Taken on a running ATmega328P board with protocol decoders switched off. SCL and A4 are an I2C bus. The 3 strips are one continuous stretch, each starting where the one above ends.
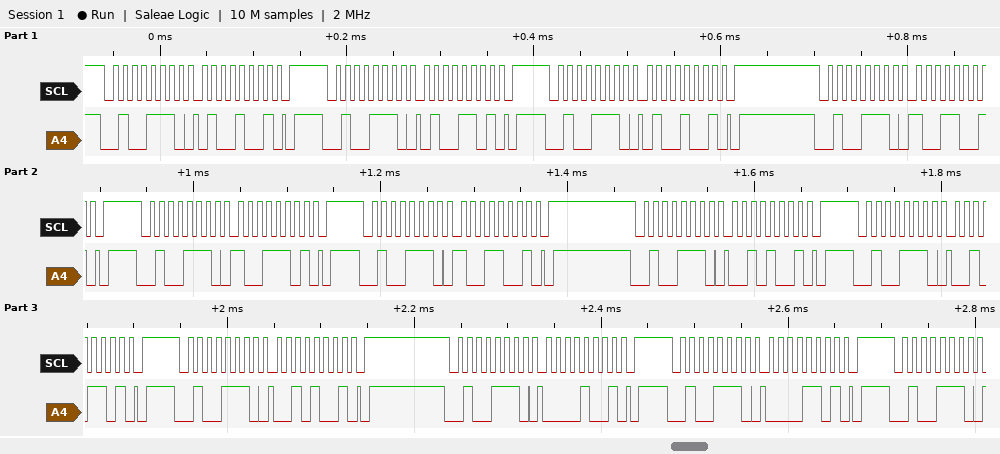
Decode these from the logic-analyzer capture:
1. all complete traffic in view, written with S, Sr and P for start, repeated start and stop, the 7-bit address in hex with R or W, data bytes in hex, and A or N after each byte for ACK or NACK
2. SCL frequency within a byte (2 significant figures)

S 27W A 49 A P S 27W A 4D A P S 27W A 49 A P S 27W A 99 A P S 27W A 9D A P S 27W A 99 A P S 27W A 29 A P S 27W A 2D A P S 27W A 29 A P S 27W A 09 A P S 27W A 0D A P S 27W A
100 kHz
